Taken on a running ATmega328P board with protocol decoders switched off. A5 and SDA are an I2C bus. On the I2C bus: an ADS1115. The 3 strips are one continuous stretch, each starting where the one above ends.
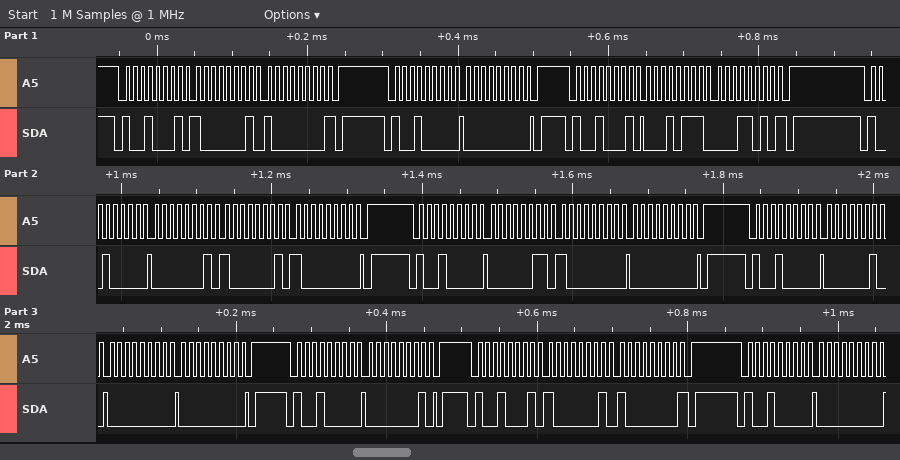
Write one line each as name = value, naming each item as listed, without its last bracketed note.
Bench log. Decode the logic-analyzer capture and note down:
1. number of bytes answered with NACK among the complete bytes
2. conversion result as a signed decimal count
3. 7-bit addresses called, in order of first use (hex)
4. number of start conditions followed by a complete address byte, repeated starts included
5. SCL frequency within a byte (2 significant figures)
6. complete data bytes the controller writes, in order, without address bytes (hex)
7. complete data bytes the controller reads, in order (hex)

number of bytes answered with NACK among the complete bytes = 3
conversion result as a signed decimal count = 5914
7-bit addresses called, in order of first use = 0x48
number of start conditions followed by a complete address byte, repeated starts included = 9
SCL frequency within a byte = 100 kHz
complete data bytes the controller writes, in order, without address bytes = 00 01 81 80 03 80 00 02 00 00 01 00
complete data bytes the controller reads, in order = 81 80 17 1A 81 80
